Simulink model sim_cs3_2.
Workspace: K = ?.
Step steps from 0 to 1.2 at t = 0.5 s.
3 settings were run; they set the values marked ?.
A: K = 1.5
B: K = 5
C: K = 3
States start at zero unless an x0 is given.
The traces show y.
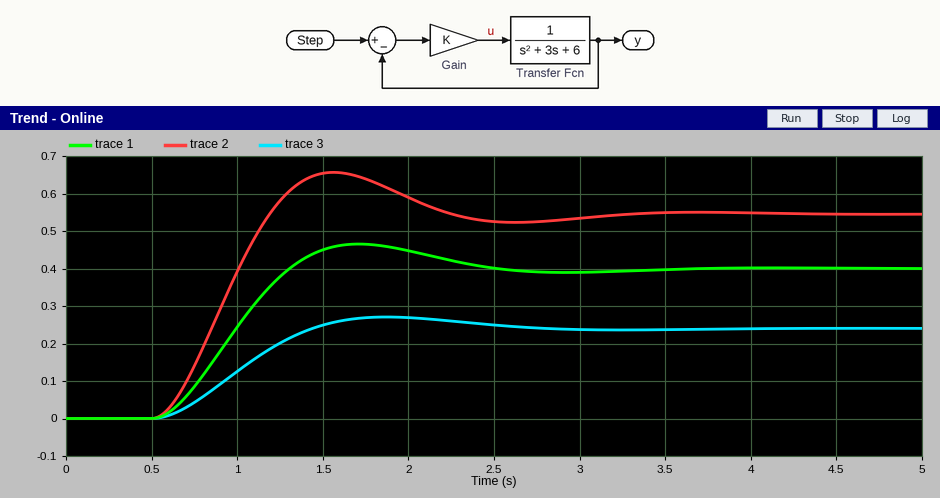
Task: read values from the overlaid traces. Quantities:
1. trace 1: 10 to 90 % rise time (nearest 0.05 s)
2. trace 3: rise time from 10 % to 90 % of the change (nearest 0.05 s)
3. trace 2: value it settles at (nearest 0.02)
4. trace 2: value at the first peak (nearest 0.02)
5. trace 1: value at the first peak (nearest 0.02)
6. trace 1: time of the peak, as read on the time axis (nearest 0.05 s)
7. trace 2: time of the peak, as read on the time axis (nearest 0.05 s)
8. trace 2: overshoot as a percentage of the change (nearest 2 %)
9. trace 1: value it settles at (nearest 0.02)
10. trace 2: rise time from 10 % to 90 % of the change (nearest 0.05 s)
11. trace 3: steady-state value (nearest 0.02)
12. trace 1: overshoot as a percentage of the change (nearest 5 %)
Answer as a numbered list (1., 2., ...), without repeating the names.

1. 0.55 s
2. 0.65 s
3. 0.54
4. 0.66
5. 0.46
6. 1.70 s
7. 1.55 s
8. 20 %
9. 0.40
10. 0.45 s
11. 0.24
12. 15 %
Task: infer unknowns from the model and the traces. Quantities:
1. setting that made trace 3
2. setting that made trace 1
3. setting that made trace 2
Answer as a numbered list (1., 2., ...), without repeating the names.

1. A
2. C
3. B
